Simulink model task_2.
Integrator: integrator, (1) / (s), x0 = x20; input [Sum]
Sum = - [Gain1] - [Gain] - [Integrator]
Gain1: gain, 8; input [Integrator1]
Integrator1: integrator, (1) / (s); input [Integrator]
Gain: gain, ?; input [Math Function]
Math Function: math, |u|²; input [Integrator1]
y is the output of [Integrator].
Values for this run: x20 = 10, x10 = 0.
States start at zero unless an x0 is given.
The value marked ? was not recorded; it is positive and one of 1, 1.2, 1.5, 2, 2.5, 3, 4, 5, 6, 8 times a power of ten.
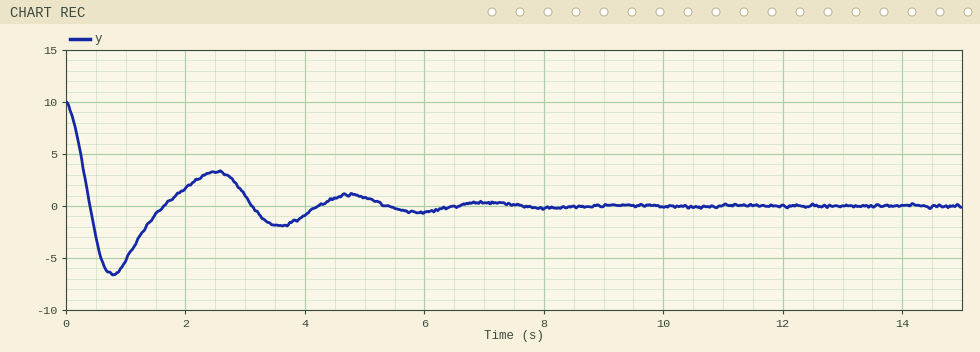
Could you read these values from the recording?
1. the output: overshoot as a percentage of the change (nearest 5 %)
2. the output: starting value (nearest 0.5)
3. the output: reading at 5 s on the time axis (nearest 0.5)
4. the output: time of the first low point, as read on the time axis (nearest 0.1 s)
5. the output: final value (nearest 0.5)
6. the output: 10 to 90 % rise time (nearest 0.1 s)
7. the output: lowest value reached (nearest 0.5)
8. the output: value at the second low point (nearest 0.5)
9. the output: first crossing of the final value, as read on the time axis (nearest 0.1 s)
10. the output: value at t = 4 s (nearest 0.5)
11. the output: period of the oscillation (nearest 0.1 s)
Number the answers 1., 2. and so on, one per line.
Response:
1. 65 %
2. 10.0
3. 1.0
4. 0.8 s
5. 0.0
6. 0.3 s
7. -6.5
8. -2.0
9. 0.4 s
10. -1.0
11. 2.8 s
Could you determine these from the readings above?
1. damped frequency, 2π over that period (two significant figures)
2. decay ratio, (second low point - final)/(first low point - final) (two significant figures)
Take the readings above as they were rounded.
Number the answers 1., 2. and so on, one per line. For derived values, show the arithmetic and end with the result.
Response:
1. 2π / 2.8 = 2.2 rad/s
2. (-2 - 0) / (-6.5 - 0) = 0.31
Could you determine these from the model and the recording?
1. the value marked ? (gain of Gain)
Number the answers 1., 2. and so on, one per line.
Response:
1. 2.5
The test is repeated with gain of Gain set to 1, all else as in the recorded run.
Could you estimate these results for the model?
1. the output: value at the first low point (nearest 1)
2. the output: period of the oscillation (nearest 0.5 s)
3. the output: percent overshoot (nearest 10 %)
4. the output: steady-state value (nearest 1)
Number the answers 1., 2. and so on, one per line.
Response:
1. -6
2. 2.5 s
3. 60 %
4. 0
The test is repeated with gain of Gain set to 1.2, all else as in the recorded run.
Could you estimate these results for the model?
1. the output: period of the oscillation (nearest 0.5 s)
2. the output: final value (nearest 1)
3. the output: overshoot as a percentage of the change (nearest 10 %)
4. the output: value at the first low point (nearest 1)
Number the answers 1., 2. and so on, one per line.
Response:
1. 2.5 s
2. 0
3. 60 %
4. -6
